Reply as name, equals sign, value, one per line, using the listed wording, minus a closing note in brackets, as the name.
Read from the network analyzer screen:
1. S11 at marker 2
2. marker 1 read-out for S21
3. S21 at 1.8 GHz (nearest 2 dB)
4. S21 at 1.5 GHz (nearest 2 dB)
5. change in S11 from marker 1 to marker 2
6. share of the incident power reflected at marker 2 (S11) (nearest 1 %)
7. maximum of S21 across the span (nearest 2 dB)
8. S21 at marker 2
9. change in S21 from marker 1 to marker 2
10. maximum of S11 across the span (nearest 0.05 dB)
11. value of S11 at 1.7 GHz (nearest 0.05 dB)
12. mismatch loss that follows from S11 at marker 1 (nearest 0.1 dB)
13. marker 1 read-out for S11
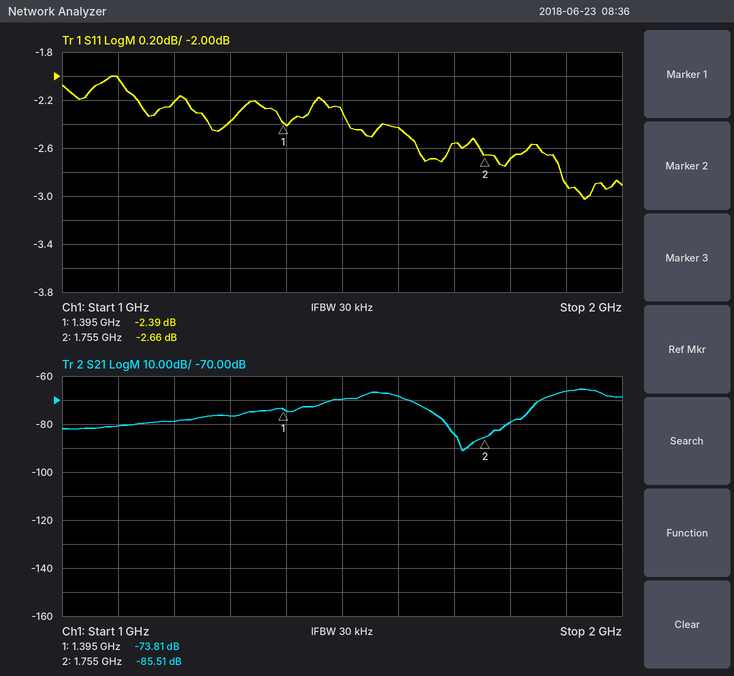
S11 at marker 2 = -2.66 dB
marker 1 read-out for S21 = -73.81 dB
S21 at 1.8 GHz = -80 dB
S21 at 1.5 GHz = -70 dB
change in S11 from marker 1 to marker 2 = -0.27 dB
share of the incident power reflected at marker 2 (S11) = 54 %
maximum of S21 across the span = -66 dB
S21 at marker 2 = -85.51 dB
change in S21 from marker 1 to marker 2 = -11.70 dB
maximum of S11 across the span = -2.00 dB
value of S11 at 1.7 GHz = -2.55 dB
mismatch loss that follows from S11 at marker 1 = 3.7 dB
marker 1 read-out for S11 = -2.39 dB
